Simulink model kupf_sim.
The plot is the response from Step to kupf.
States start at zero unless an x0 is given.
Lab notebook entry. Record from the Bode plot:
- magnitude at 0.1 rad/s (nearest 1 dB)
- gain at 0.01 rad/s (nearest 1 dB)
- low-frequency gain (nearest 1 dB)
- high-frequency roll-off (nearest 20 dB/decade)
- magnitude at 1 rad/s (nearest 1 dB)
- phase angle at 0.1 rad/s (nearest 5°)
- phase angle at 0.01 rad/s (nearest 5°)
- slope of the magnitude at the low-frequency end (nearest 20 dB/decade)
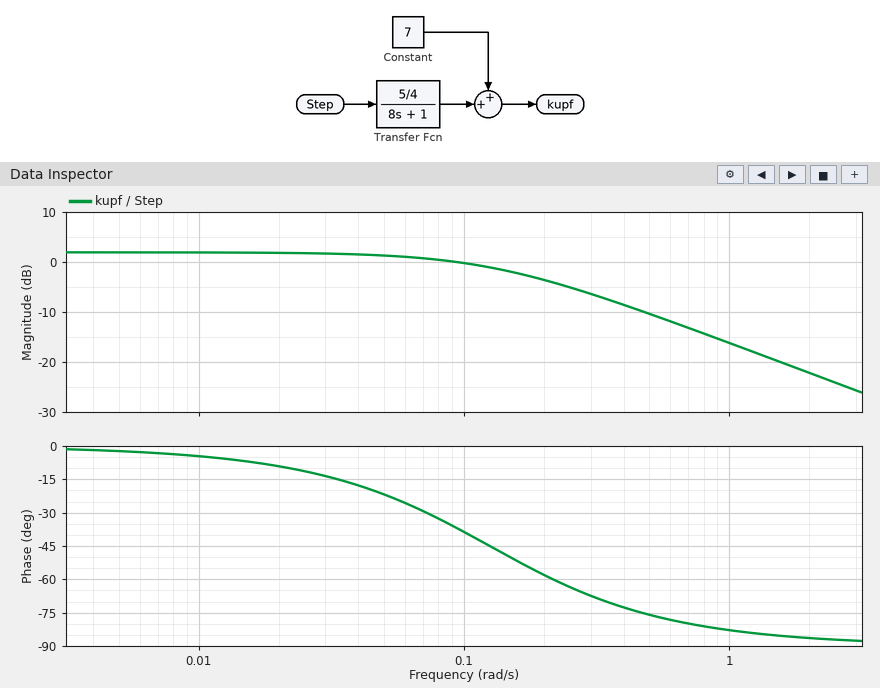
0 dB
2 dB
2 dB
-20 dB/decade
-16 dB
-40°
-5°
0 dB/decade
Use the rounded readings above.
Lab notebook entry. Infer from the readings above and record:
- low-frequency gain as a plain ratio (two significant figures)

1.3
